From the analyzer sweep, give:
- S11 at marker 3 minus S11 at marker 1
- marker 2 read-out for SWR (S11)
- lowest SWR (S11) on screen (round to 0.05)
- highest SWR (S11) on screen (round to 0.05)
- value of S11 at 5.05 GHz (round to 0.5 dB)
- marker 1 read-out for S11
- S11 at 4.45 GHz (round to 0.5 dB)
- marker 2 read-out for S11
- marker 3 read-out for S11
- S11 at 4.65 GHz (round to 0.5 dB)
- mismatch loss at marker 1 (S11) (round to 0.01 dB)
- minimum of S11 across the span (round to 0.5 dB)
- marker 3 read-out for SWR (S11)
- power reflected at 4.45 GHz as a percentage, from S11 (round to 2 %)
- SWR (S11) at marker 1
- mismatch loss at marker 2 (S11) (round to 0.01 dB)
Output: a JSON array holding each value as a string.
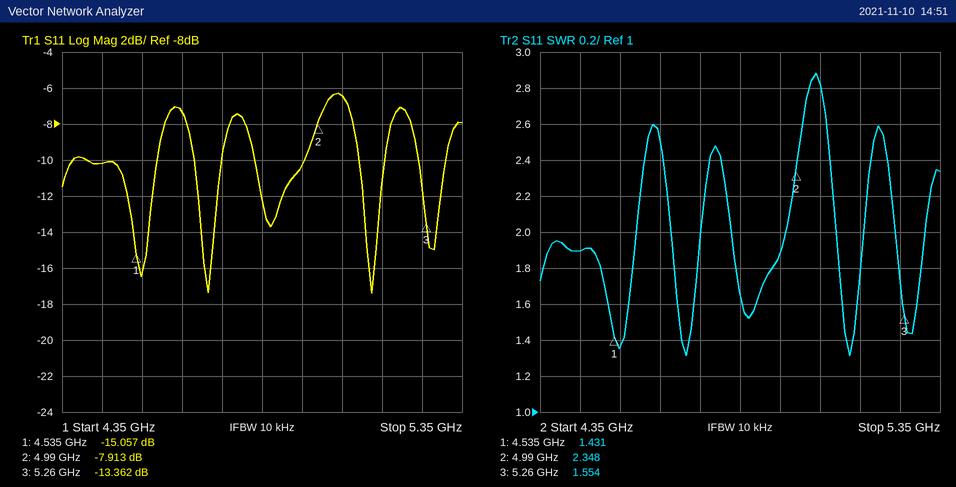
["1.695 dB", "2.348", "1.30", "2.90", "-6.5 dB", "-15.057 dB", "-10.0 dB", "-7.913 dB", "-13.362 dB", "-7.5 dB", "0.14 dB", "-17.5 dB", "1.554", "10 %", "1.431", "0.77 dB"]
